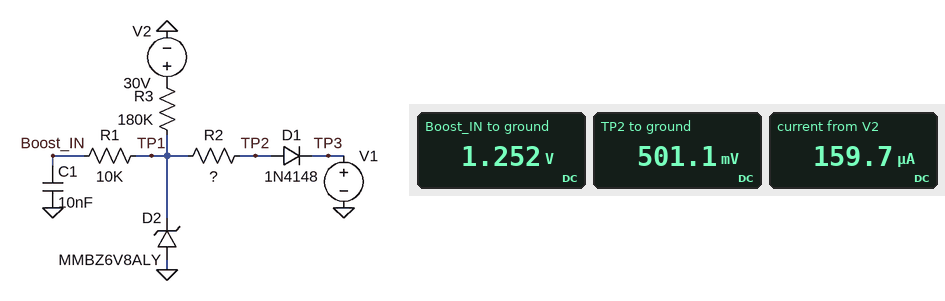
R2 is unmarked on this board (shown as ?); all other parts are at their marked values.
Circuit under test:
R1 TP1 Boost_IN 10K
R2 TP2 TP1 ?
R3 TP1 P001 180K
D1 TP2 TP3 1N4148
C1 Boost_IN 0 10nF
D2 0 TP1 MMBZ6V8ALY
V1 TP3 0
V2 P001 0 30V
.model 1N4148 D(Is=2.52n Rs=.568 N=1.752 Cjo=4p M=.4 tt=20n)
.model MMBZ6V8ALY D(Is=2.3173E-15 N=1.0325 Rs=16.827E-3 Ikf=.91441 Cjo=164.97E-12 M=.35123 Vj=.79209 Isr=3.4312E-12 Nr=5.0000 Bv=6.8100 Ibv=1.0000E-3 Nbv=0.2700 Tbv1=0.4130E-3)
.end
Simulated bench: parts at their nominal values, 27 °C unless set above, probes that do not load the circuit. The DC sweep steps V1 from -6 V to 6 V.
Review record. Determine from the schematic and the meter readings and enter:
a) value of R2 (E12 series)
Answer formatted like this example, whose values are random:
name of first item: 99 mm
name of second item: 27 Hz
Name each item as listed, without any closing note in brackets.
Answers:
value of R2: 4.7 kΩ
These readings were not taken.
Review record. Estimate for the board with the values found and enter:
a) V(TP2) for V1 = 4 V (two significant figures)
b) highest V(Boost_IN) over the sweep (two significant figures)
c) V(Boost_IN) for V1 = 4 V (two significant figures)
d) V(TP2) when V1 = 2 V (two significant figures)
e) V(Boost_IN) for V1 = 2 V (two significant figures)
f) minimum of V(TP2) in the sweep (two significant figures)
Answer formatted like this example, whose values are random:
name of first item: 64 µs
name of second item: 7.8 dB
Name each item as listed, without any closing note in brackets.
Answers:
V(TP2) for V1 = 4 V: 4.5 V
highest V(Boost_IN) over the sweep: 6.8 V
V(Boost_IN) for V1 = 4 V: 5.1 V
V(TP2) when V1 = 2 V: 2.5 V
V(Boost_IN) for V1 = 2 V: 3.2 V
minimum of V(TP2) in the sweep: -5.4 V
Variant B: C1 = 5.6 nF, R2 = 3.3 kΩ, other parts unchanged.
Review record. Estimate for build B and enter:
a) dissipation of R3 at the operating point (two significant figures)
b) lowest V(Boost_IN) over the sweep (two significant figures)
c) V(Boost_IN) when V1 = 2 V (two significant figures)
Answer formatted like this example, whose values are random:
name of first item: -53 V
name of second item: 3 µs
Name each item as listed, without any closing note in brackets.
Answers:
dissipation of R3 at the operating point: 4.7 mW
lowest V(Boost_IN) over the sweep: -720 mV
V(Boost_IN) when V1 = 2 V: 3.0 V
